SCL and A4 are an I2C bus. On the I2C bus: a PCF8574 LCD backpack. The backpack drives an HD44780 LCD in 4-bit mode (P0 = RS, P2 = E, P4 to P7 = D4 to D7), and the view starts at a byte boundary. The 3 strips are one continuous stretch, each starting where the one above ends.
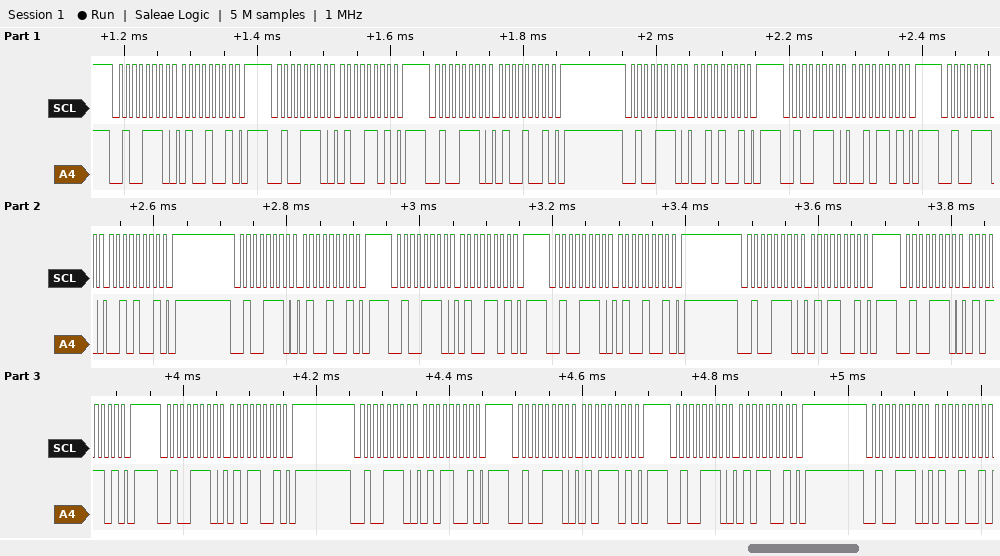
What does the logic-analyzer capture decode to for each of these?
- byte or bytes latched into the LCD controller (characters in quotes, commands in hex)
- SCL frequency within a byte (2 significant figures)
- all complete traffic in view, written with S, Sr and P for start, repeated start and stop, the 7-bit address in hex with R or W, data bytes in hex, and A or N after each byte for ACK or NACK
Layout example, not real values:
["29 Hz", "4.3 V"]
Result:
["'B' 'E'", "100 kHz", "S 27W A 49 A P S 27W A 4D A P S 27W A 49 A P S 27W A 29 A P S 27W A 2D A P S 27W A 29 A P S 27W A 49 A P S 27W A 4D A P S 27W A 49 A P S 27W A 59 A P S 27W A 5D A P S 27W A 59 A P S 27W A 59 A P S 27W A 5D A P S 27W A 59 A P S 27W A 49 A"]
